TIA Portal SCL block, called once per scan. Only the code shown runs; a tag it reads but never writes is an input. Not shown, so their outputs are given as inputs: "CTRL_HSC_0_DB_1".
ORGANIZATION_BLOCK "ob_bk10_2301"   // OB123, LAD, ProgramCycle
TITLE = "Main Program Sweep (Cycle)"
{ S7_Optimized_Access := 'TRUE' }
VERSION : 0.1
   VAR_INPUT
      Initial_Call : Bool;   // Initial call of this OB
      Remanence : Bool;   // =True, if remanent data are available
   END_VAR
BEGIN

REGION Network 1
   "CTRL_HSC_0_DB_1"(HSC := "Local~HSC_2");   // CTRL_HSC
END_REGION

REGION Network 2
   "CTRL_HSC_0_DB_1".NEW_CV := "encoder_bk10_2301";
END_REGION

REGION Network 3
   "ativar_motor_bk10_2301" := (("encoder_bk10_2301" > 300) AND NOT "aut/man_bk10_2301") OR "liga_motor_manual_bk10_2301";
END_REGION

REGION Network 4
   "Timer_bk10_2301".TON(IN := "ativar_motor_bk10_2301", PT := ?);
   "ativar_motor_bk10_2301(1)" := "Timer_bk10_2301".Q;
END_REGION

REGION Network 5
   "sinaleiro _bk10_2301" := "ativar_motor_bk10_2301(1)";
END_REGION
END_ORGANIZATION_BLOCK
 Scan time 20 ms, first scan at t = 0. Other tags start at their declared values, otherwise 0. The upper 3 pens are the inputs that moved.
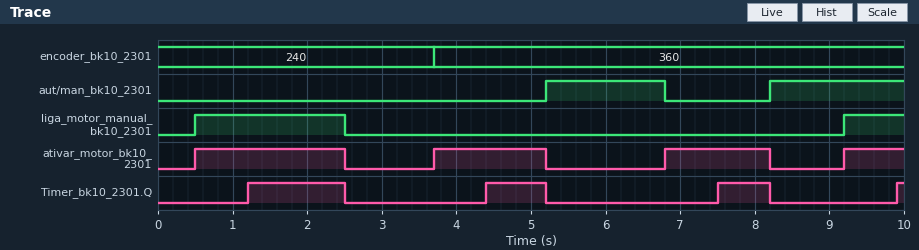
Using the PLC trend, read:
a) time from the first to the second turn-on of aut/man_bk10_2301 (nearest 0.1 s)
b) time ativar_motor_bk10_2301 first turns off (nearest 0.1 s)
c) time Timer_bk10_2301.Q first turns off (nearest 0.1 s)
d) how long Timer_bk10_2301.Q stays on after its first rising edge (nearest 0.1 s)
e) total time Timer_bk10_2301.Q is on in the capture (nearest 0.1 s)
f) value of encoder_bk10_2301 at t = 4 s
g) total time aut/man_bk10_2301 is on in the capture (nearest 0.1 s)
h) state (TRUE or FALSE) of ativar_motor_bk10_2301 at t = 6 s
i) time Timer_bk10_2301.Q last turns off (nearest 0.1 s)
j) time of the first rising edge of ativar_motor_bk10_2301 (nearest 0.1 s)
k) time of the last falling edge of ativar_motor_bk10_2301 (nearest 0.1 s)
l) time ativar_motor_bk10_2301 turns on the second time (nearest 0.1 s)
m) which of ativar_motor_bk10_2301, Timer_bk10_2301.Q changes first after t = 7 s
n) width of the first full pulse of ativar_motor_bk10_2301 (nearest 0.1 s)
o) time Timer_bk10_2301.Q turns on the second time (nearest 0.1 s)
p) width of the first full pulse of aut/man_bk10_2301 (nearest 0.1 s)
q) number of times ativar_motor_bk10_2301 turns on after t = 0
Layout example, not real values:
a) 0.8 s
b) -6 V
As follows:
a) 3.0 s
b) 2.5 s
c) 2.5 s
d) 1.3 s
e) 2.9 s
f) 360
g) 3.4 s
h) FALSE
i) 8.2 s
j) 0.5 s
k) 8.2 s
l) 3.7 s
m) Timer_bk10_2301.Q
n) 2.0 s
o) 4.4 s
p) 1.6 s
q) 4
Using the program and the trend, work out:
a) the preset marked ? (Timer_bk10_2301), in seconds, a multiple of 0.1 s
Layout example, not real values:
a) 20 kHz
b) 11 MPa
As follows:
a) 0.7 s
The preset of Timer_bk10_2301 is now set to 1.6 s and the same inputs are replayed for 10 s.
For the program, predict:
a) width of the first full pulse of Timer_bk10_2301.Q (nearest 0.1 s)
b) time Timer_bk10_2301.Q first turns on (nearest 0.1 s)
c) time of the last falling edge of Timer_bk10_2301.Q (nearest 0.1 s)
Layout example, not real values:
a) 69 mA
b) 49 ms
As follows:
a) 0.4 s
b) 2.1 s
c) 2.5 s
